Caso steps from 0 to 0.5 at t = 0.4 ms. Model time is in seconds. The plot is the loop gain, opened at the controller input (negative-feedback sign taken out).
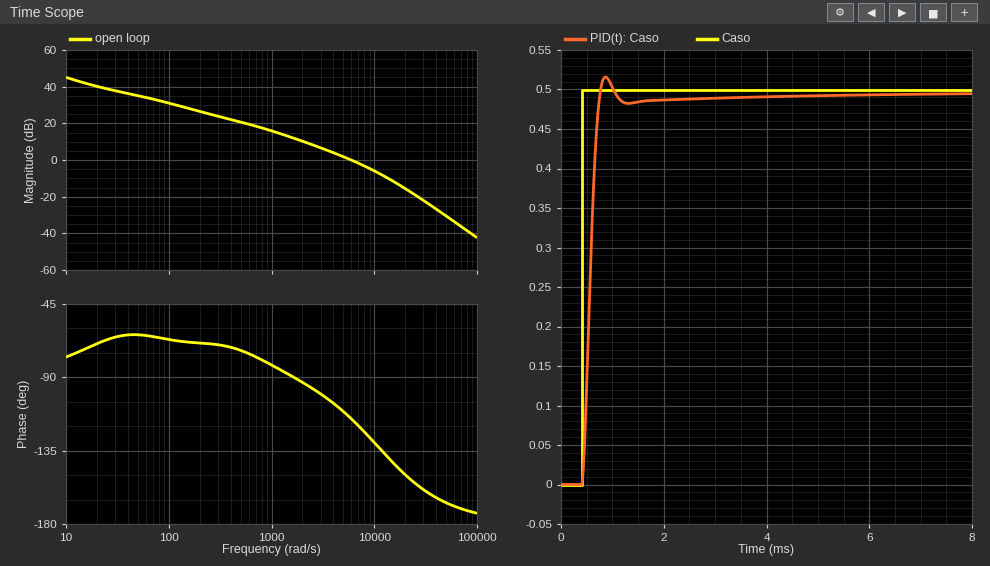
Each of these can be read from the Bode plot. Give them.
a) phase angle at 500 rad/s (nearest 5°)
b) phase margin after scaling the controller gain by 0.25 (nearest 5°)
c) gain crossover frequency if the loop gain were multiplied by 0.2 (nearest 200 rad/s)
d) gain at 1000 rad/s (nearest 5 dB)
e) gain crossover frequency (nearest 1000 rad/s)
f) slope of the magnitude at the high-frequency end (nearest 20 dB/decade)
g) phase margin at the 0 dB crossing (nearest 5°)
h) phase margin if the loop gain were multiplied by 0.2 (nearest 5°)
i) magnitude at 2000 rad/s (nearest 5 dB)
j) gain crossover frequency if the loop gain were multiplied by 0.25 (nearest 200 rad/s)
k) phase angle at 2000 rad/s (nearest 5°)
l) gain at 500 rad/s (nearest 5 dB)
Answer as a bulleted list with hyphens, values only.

- -75°
- 90°
- 1200 rad/s
- 15 dB
- 6000 rad/s
- -40 dB/decade
- 65°
- 95°
- 10 dB
- 1600 rad/s
- -95°
- 20 dB
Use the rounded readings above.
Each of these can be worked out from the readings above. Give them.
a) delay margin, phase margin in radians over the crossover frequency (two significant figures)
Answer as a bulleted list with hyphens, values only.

- 0.00019 s
